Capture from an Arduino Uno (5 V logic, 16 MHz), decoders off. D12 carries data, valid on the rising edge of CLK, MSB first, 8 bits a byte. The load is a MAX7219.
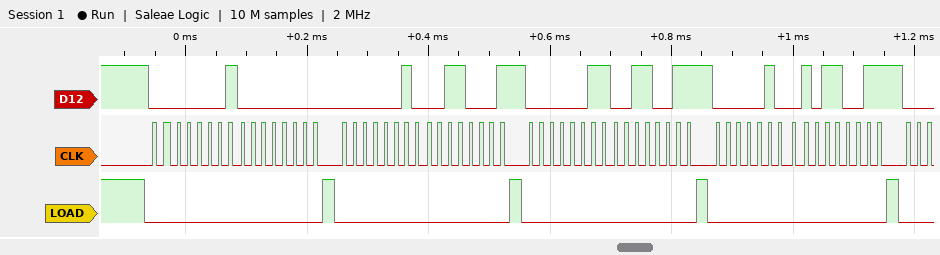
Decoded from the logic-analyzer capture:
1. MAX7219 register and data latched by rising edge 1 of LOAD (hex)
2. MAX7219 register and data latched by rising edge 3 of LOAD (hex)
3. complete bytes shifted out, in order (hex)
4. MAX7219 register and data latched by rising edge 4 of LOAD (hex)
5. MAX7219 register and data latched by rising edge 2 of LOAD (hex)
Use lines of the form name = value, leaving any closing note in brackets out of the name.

MAX7219 register and data latched by rising edge 1 of LOAD = register 0x1, data 0x00
MAX7219 register and data latched by rising edge 3 of LOAD = register 0x3, data 0x33
complete bytes shifted out, in order = 0x01 0x00 0x02 0x31 0x03 0x33 0x04 0xB3
MAX7219 register and data latched by rising edge 4 of LOAD = register 0x4, data 0xB3
MAX7219 register and data latched by rising edge 2 of LOAD = register 0x2, data 0x31
